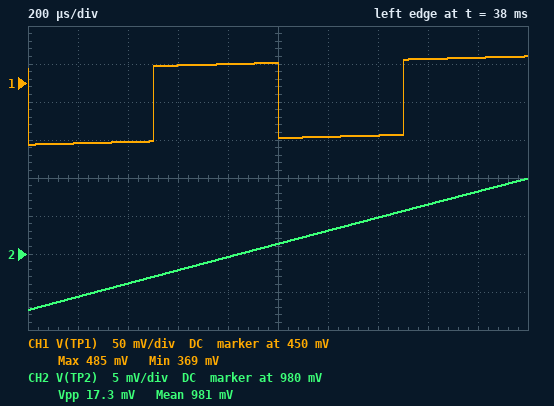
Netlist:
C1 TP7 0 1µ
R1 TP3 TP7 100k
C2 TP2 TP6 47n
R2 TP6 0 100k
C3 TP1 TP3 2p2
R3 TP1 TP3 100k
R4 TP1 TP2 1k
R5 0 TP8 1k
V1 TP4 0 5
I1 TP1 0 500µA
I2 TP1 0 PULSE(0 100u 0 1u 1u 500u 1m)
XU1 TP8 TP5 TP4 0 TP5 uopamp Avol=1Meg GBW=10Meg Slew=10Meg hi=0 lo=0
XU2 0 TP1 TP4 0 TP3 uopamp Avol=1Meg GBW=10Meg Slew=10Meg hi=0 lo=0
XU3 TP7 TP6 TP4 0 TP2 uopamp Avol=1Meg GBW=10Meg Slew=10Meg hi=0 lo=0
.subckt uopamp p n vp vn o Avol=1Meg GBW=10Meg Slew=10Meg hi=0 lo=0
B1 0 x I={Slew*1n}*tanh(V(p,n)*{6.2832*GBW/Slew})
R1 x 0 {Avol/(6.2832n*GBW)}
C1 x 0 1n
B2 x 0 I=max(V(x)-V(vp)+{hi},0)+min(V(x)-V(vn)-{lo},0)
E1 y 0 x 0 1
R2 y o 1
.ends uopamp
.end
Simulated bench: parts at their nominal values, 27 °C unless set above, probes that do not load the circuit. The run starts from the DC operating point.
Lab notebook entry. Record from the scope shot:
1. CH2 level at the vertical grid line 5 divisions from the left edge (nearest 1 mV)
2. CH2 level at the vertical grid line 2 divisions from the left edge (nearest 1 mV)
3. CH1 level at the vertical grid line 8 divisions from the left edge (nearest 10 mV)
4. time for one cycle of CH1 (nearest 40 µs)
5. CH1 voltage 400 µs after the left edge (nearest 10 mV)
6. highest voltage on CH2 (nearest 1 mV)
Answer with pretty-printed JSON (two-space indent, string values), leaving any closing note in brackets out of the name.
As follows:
{
  "CH2 level at the vertical grid line 5 divisions from the left edge": "981 mV",
  "CH2 level at the vertical grid line 2 divisions from the left edge": "976 mV",
  "CH1 level at the vertical grid line 8 divisions from the left edge": "480 mV",
  "time for one cycle of CH1": "1.00 ms",
  "CH1 voltage 400 µs after the left edge": "370 mV",
  "highest voltage on CH2": "990 mV"
}
